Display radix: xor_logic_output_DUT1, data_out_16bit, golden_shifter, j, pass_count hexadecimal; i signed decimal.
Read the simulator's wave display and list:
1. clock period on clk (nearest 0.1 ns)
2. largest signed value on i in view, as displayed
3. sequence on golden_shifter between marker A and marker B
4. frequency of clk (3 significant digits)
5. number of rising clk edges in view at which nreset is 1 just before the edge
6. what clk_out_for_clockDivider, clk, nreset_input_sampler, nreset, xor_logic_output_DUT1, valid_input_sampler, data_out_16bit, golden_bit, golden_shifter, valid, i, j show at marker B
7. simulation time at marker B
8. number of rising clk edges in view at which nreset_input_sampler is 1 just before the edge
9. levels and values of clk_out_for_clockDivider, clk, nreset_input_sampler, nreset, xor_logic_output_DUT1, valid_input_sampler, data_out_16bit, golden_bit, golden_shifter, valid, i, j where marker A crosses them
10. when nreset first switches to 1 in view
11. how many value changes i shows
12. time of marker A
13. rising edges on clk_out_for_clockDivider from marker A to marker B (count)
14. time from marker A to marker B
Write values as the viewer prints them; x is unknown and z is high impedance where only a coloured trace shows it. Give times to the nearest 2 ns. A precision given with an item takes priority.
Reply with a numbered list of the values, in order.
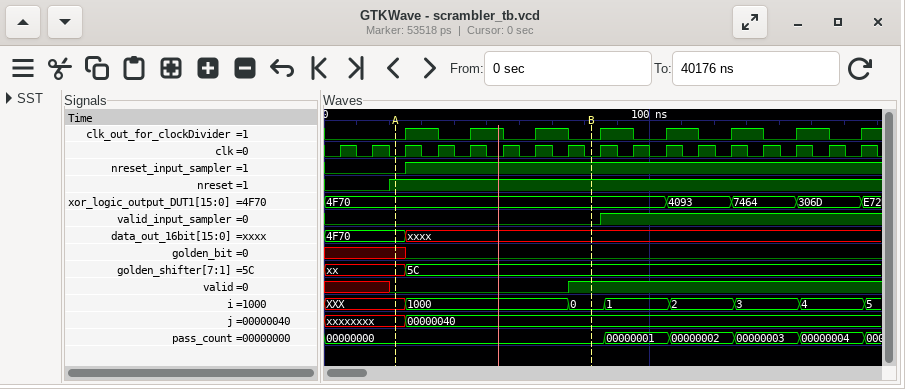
1. 10 ns
2. 1000
3. xx, 5C
4. 100 MHz
5. 15
6. clk_out_for_clockDivider=0, clk=0, nreset_input_sampler=1, nreset=1, xor_logic_output_DUT1=4F70, valid_input_sampler=0, data_out_16bit=xxxx, golden_bit=0, golden_shifter=5C, valid=1, i=0, j=00000040
7. 82 ns
8. 14
9. clk_out_for_clockDivider=0, clk=0, nreset_input_sampler=0, nreset=1, xor_logic_output_DUT1=4F70, valid_input_sampler=0, data_out_16bit=4F70, golden_bit=x, golden_shifter=xx, valid=0, i=XXX, j=xxxxxxxx
10. 20 ns
11. 7
12. 22 ns
13. 3
14. 60 ns
